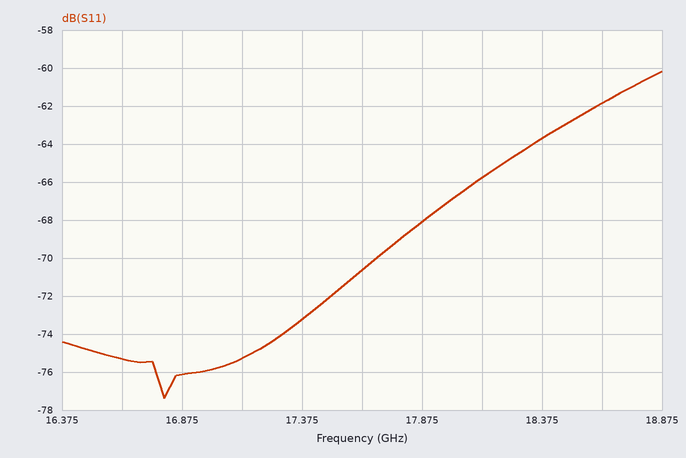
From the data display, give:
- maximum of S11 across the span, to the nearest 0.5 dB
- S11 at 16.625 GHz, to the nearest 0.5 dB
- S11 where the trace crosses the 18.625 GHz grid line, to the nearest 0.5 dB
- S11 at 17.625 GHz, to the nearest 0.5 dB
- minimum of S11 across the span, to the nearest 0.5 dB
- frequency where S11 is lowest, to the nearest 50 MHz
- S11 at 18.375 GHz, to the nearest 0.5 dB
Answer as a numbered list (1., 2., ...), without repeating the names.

1. -60.0 dB
2. -75.5 dB
3. -62.0 dB
4. -70.5 dB
5. -77.5 dB
6. 16.80 GHz
7. -63.5 dB
